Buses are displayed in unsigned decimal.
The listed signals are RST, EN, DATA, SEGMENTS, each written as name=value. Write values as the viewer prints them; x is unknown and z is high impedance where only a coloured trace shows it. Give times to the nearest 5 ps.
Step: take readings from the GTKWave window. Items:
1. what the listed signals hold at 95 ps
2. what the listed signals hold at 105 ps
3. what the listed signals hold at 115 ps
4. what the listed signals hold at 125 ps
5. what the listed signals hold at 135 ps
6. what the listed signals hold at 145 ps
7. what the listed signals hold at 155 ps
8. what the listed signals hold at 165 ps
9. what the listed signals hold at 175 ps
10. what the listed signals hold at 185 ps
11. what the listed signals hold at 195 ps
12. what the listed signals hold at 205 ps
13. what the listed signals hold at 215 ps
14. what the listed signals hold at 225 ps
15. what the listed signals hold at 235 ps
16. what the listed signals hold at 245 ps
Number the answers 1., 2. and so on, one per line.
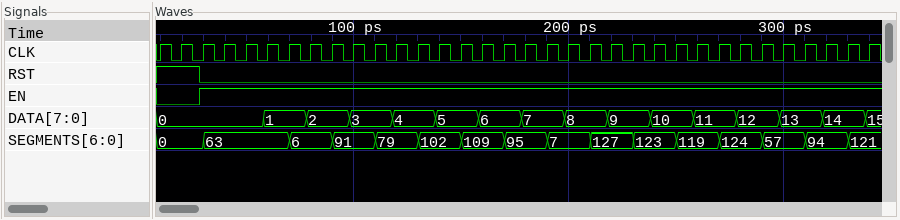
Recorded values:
1. RST=0, EN=1, DATA=2, SEGMENTS=91
2. RST=0, EN=1, DATA=3, SEGMENTS=91
3. RST=0, EN=1, DATA=3, SEGMENTS=79
4. RST=0, EN=1, DATA=4, SEGMENTS=79
5. RST=0, EN=1, DATA=4, SEGMENTS=102
6. RST=0, EN=1, DATA=5, SEGMENTS=102
7. RST=0, EN=1, DATA=5, SEGMENTS=109
8. RST=0, EN=1, DATA=6, SEGMENTS=109
9. RST=0, EN=1, DATA=6, SEGMENTS=95
10. RST=0, EN=1, DATA=7, SEGMENTS=95
11. RST=0, EN=1, DATA=7, SEGMENTS=7
12. RST=0, EN=1, DATA=8, SEGMENTS=7
13. RST=0, EN=1, DATA=8, SEGMENTS=127
14. RST=0, EN=1, DATA=9, SEGMENTS=127
15. RST=0, EN=1, DATA=9, SEGMENTS=123
16. RST=0, EN=1, DATA=10, SEGMENTS=123
